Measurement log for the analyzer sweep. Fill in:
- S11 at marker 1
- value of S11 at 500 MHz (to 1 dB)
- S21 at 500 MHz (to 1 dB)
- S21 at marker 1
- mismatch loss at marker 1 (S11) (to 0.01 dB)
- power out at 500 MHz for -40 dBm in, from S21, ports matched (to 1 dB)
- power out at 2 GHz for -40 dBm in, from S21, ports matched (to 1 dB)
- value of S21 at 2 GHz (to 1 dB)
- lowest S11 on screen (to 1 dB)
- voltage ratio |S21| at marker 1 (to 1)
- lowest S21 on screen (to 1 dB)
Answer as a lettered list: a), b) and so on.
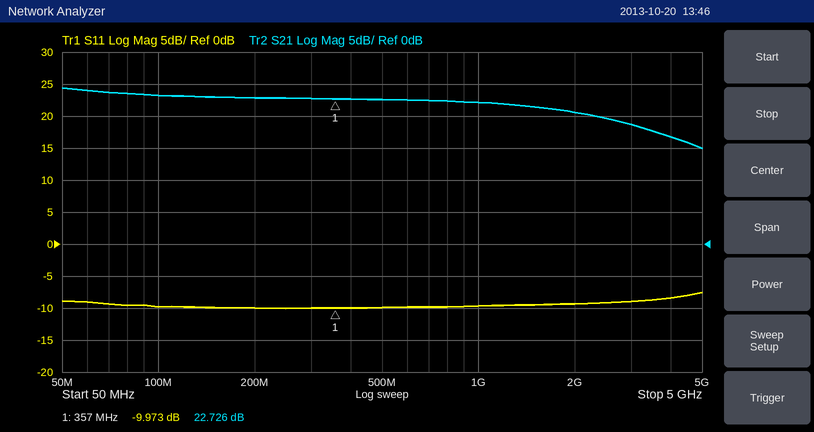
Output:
a) -9.973 dB
b) -10 dB
c) 23 dB
d) 22.726 dB
e) 0.46 dB
f) -17 dBm
g) -19 dBm
h) 21 dB
i) -10 dB
j) 14
k) 15 dB
